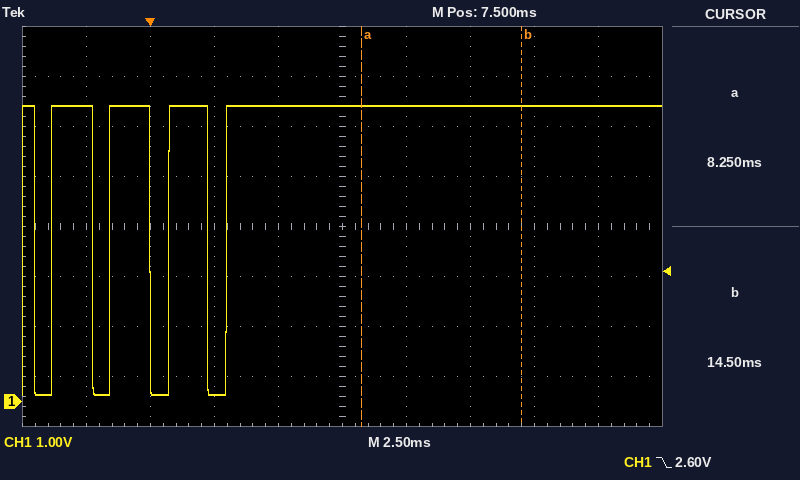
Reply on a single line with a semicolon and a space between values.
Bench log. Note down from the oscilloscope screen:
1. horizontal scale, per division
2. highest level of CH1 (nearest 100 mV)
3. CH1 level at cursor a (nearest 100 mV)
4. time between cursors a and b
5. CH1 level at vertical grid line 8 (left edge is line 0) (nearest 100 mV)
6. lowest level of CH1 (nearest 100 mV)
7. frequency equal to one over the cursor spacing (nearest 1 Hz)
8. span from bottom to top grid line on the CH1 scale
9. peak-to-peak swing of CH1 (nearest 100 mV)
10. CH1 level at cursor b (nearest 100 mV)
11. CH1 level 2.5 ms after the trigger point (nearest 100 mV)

2.5 ms; 5.9 V; 5.9 V; 6.25 ms; 5.9 V; 100 mV; 160 Hz; 8 V; 5.8 V; 5.9 V; 100 mV
